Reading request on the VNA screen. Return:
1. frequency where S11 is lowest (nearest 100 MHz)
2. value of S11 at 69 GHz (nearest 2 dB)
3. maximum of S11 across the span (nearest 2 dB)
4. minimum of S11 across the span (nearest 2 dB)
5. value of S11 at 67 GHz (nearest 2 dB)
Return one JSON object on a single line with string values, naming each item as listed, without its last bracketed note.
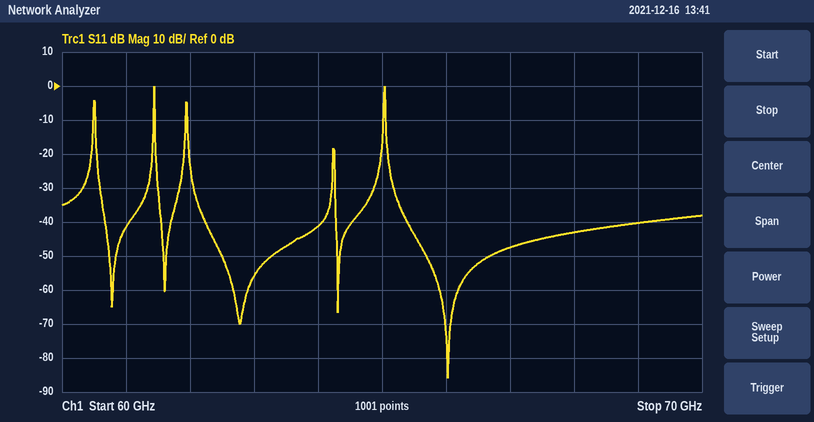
{"frequency where S11 is lowest": "66.0 GHz", "value of S11 at 69 GHz": "-40 dB", "maximum of S11 across the span": "0 dB", "minimum of S11 across the span": "-86 dB", "value of S11 at 67 GHz": "-48 dB"}
